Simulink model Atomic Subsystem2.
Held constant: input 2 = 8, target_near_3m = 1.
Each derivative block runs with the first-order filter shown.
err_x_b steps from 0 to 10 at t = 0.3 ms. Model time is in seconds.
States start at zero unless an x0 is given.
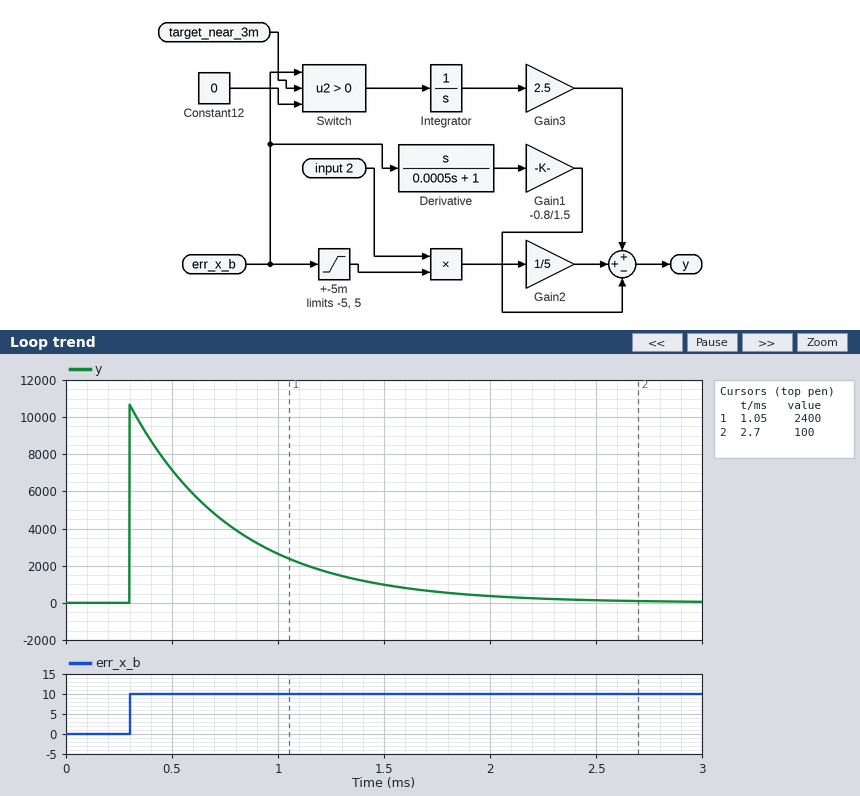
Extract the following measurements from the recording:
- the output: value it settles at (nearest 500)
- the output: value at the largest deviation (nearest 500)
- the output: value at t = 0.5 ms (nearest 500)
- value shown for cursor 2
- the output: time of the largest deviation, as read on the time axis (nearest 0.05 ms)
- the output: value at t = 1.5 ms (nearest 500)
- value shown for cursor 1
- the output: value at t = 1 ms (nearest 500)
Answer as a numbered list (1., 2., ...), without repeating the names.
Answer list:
1. 0
2. 10500
3. 7000
4. 100
5. 0.30 ms
6. 1000
7. 2400
8. 2500
